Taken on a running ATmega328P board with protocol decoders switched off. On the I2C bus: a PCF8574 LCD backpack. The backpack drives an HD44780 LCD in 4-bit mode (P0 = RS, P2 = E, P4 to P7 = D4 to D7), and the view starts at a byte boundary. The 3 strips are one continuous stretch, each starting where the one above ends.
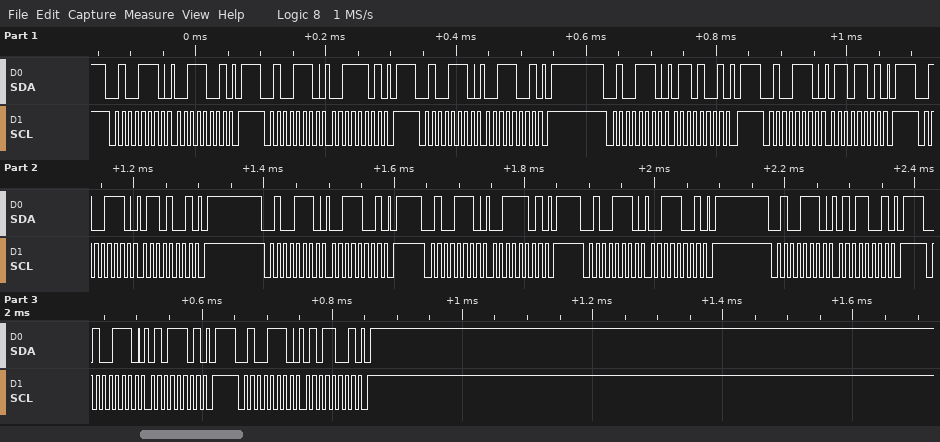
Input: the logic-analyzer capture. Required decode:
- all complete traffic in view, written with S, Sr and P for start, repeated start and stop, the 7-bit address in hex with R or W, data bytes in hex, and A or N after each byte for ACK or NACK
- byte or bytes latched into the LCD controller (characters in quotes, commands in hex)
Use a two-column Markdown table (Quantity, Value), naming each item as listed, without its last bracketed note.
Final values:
| Quantity | Value |
|---|---|
| all complete traffic in view, written with S, Sr and P for start, repeated start and stop, the 7-bit address in hex with R or W, data bytes in hex, and A or N after each byte for ACK or NACK | S 27W A 39 A P S 27W A 3D A P S 27W A 39 A P S 27W A 69 A P S 27W A 6D A P S 27W A 69 A P S 27W A 39 A P S 27W A 3D A P S 27W A 39 A P S 27W A 59 A P S 27W A 5D A P S 27W A 59 A P |
| byte or bytes latched into the LCD controller | '6' '5' |
